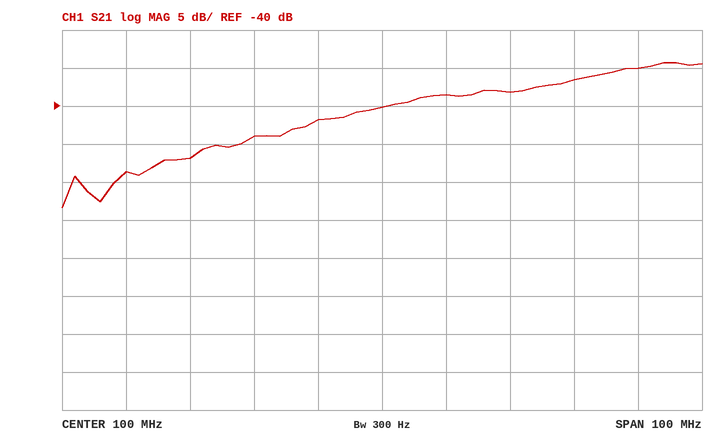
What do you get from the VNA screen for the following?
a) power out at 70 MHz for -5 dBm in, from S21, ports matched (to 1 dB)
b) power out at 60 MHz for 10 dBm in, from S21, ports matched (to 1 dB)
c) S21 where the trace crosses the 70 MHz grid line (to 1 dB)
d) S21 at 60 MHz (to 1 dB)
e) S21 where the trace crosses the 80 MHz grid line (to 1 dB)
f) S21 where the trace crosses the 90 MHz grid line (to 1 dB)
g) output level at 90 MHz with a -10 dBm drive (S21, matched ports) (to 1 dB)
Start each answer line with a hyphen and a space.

- -52 dBm
- -39 dBm
- -47 dB
- -49 dB
- -44 dB
- -42 dB
- -52 dBm
